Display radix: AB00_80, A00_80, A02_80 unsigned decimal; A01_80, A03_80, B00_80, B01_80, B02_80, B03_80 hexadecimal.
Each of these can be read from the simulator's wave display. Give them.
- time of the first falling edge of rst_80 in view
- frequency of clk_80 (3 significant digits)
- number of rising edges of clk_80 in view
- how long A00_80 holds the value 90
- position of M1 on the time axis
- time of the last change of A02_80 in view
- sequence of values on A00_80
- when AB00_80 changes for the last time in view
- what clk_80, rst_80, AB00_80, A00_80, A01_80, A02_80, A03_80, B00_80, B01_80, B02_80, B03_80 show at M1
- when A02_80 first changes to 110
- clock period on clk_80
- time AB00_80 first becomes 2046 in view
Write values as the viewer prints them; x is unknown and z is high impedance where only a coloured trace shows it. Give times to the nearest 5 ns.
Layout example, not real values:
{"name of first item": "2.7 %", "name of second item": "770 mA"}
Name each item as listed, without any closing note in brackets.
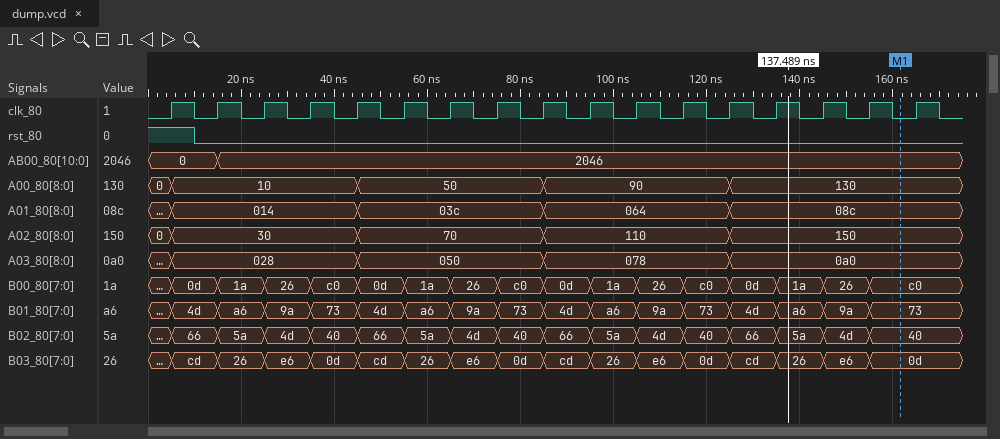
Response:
{"time of the first falling edge of rst_80 in view": "10 ns", "frequency of clk_80": "100 MHz", "number of rising edges of clk_80 in view": "17", "how long A00_80 holds the value 90": "40 ns", "position of M1 on the time axis": "160 ns", "time of the last change of A02_80 in view": "125 ns", "sequence of values on A00_80": "0, 10, 50, 90, 130", "when AB00_80 changes for the last time in view": "15 ns", "what clk_80, rst_80, AB00_80, A00_80, A01_80, A02_80, A03_80, B00_80, B01_80, B02_80, B03_80 show at M1": "clk_80=0, rst_80=0, AB00_80=2046, A00_80=130, A01_80=08c, A02_80=150, A03_80=0a0, B00_80=c0, B01_80=73, B02_80=40, B03_80=0d", "when A02_80 first changes to 110": "85 ns", "clock period on clk_80": "10 ns", "time AB00_80 first becomes 2046 in view": "15 ns"}
